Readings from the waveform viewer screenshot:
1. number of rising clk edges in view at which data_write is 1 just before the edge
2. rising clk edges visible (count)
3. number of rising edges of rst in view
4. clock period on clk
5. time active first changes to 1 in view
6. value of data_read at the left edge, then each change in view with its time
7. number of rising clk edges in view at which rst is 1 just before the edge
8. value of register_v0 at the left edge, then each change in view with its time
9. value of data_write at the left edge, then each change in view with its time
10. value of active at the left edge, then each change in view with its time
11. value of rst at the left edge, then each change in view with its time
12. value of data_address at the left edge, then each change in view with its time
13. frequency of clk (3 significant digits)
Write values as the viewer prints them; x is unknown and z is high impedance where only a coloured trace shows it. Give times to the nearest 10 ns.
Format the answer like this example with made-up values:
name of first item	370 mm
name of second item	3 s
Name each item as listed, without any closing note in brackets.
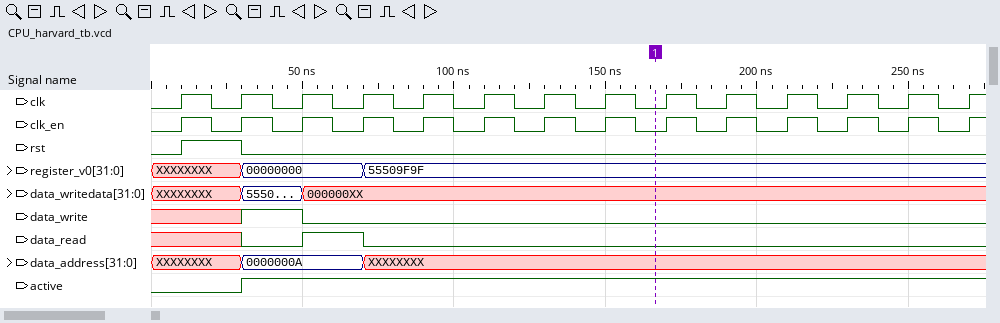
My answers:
number of rising clk edges in view at which data_write is 1 just before the edge	1
rising clk edges visible	14
number of rising edges of rst in view	1
clock period on clk	20 ns
time active first changes to 1 in view	30 ns
value of data_read at the left edge, then each change in view with its time	x, 0 at 30 ns, 1 at 50 ns, 0 at 70 ns
number of rising clk edges in view at which rst is 1 just before the edge	1
value of register_v0 at the left edge, then each change in view with its time	XXXXXXXX, 00000000 at 30 ns, 55509F9F at 70 ns
value of data_write at the left edge, then each change in view with its time	x, 1 at 30 ns, 0 at 50 ns
value of active at the left edge, then each change in view with its time	0, 1 at 30 ns
value of rst at the left edge, then each change in view with its time	0, 1 at 10 ns, 0 at 30 ns
value of data_address at the left edge, then each change in view with its time	XXXXXXXX, 0000000A at 30 ns, XXXXXXXX at 70 ns
frequency of clk	50.0 MHz
